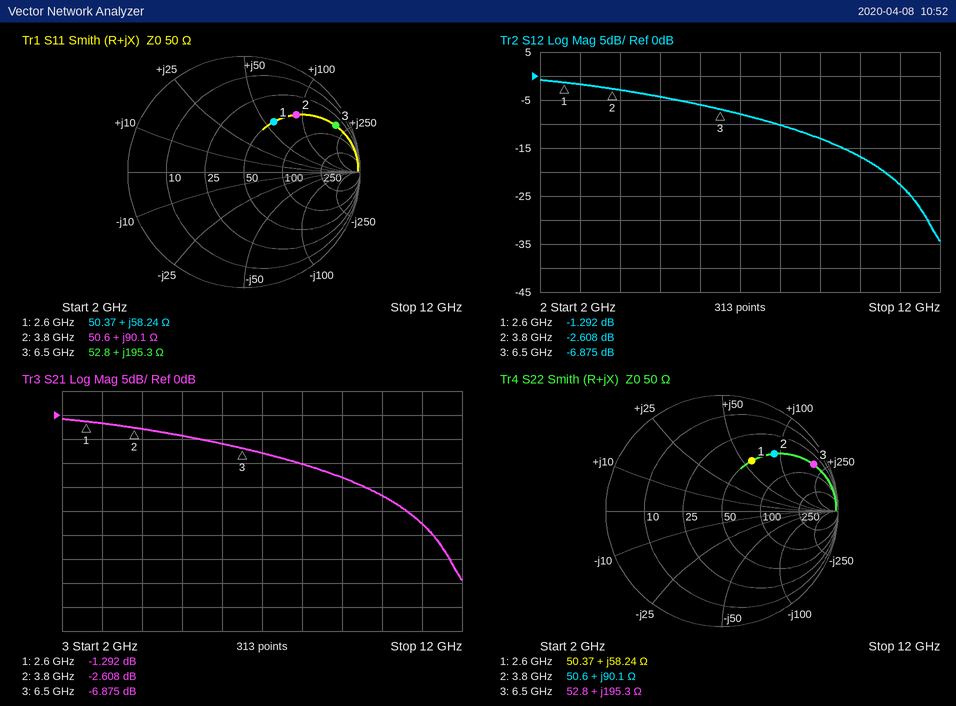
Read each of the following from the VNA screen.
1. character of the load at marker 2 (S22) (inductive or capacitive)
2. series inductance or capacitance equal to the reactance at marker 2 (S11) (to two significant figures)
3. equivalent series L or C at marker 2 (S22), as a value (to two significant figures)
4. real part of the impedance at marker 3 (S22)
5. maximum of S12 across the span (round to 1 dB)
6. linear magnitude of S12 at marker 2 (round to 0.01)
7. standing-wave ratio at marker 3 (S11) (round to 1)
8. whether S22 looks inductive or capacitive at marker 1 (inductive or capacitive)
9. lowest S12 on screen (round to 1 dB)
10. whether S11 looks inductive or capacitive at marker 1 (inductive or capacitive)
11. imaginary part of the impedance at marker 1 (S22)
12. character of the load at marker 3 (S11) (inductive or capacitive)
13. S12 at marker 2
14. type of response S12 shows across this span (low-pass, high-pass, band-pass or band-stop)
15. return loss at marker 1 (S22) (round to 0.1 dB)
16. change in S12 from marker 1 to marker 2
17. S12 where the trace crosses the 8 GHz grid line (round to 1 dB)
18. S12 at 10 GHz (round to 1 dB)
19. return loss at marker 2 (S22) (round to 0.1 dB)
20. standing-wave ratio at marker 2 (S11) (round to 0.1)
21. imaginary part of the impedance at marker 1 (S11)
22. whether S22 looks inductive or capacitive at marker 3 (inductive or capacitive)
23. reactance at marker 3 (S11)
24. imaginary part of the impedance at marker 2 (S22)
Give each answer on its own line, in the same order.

inductive
3.8 nH
3.8 nH
52.8 Ω
-1 dB
0.74
16
inductive
-34 dB
inductive
+58.24 Ω
inductive
-2.608 dB
low-pass
6.0 dB
-1.316 dB
-10 dB
-17 dB
3.5 dB
5.0
+58.24 Ω
inductive
+195.3 Ω
+90.1 Ω
